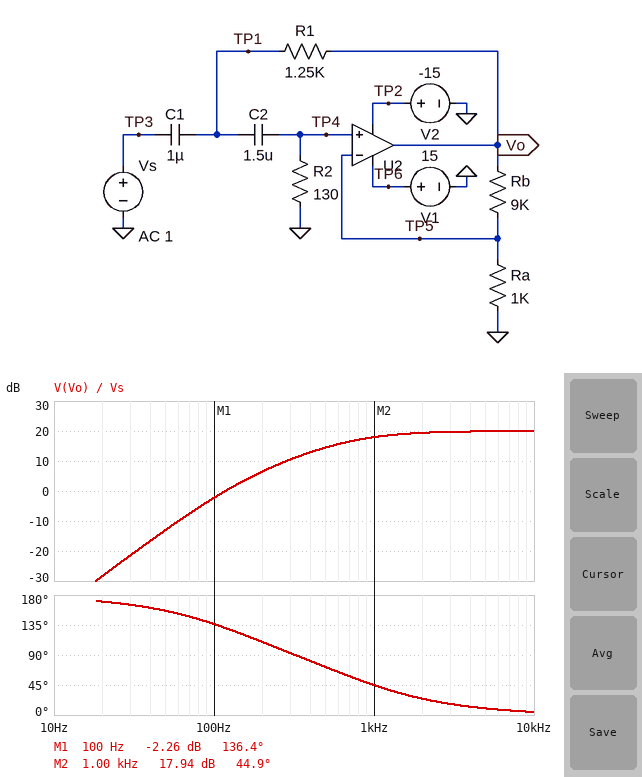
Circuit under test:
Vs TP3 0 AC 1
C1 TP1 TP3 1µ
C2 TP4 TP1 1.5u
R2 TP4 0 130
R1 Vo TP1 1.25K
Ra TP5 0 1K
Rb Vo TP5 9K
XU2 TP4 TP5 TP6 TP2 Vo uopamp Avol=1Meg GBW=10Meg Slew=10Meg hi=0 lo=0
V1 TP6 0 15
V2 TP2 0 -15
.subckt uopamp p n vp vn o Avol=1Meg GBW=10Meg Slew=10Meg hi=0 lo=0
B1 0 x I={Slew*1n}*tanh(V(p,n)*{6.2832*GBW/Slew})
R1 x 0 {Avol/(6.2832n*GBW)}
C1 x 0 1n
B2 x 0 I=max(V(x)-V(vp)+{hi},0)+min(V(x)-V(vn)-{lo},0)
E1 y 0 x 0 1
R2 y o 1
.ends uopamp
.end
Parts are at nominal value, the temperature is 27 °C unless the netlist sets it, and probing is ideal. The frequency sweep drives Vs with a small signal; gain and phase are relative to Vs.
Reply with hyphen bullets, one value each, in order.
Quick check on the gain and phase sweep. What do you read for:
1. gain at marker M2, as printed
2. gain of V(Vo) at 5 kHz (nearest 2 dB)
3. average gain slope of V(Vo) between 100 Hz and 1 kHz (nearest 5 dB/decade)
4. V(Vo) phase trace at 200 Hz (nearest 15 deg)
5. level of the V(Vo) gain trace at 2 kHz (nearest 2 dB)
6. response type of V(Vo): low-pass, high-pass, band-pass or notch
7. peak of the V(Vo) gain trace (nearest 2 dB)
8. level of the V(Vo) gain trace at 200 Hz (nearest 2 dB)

- 17.94 dB
- 20 dB
- 20 dB/decade
- 105 deg
- 20 dB
- high-pass
- 20 dB
- 6 dB
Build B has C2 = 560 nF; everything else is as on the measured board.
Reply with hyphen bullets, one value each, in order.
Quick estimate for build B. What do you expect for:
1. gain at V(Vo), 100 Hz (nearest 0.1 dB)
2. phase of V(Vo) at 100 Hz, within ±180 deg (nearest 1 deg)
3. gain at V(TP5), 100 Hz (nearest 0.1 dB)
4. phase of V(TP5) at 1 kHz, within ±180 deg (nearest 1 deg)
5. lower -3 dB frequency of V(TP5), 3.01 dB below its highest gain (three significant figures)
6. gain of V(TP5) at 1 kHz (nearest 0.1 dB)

- -10.9 dB
- 140 deg
- -30.9 dB
- 72 deg
- 2.13 kHz
- -7.5 dB
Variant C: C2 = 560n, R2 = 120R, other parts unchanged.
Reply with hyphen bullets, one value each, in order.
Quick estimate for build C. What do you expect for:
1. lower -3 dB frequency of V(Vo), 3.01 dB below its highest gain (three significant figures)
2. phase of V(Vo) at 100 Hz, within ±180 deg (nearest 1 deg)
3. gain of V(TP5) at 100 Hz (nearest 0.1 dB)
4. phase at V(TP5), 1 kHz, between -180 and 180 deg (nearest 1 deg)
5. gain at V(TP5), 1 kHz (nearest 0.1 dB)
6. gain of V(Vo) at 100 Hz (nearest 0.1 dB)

- 2.42 kHz
- 139 deg
- -31.8 dB
- 75 deg
- -8.4 dB
- -11.8 dB
